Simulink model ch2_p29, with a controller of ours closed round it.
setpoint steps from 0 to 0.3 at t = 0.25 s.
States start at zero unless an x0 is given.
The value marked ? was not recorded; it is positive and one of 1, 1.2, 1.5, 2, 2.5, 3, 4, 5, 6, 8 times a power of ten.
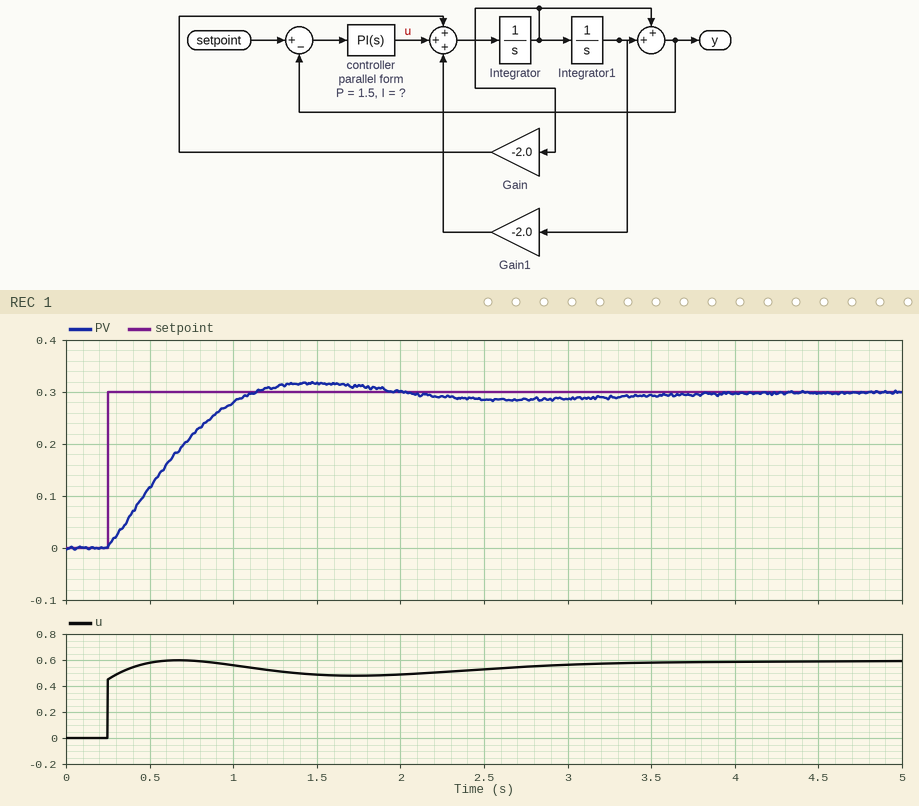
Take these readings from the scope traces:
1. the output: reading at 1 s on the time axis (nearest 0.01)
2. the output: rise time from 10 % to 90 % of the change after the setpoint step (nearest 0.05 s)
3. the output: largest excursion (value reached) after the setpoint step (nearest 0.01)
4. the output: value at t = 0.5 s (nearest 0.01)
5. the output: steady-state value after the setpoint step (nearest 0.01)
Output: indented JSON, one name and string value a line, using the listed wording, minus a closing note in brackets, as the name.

{
  "the output: reading at 1 s on the time axis": "0.28",
  "the output: rise time from 10 % to 90 % of the change after the setpoint step": "0.65 s",
  "the output: largest excursion (value reached) after the setpoint step": "0.32",
  "the output: value at t = 0.5 s": "0.12",
  "the output: steady-state value after the setpoint step": "0.30"
}
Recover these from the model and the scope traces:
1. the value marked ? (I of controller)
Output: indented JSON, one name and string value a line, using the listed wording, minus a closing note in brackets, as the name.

{
  "the value marked ?": "5"
}
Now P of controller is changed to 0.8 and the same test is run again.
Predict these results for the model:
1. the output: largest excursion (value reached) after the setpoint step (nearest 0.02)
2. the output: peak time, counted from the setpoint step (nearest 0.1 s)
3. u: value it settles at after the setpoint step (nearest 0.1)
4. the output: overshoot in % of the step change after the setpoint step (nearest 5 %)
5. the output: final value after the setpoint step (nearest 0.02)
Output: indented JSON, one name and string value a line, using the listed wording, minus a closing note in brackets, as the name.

{
  "the output: largest excursion (value reached) after the setpoint step": "0.34",
  "the output: peak time, counted from the setpoint step": "1.3 s",
  "u: value it settles at after the setpoint step": "0.6",
  "the output: overshoot in % of the step change after the setpoint step": "15 %",
  "the output: final value after the setpoint step": "0.30"
}
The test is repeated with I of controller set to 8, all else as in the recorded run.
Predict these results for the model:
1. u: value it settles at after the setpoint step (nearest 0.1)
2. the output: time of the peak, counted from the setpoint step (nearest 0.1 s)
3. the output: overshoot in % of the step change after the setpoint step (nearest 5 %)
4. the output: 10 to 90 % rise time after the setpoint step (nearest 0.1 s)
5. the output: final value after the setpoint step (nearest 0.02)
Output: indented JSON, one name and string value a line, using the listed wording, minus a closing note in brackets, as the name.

{
  "u: value it settles at after the setpoint step": "0.6",
  "the output: time of the peak, counted from the setpoint step": "1.0 s",
  "the output: overshoot in % of the step change after the setpoint step": "15 %",
  "the output: 10 to 90 % rise time after the setpoint step": "0.5 s",
  "the output: final value after the setpoint step": "0.30"
}
